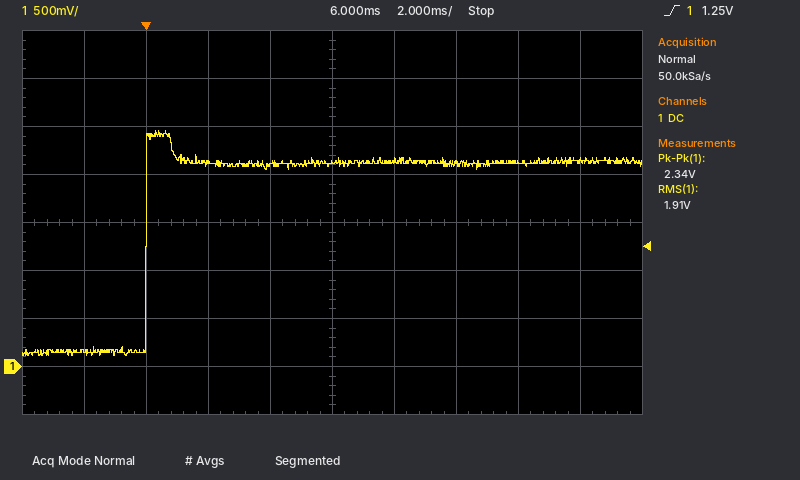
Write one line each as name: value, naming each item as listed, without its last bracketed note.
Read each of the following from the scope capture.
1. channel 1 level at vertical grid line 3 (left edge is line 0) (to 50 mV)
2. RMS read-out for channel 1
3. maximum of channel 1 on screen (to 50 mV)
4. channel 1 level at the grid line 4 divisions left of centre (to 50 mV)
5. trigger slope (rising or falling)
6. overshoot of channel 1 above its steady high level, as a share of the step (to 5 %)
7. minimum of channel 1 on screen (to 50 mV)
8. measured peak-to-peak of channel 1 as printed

channel 1 level at vertical grid line 3 (left edge is line 0): 2.10 V
RMS read-out for channel 1: 1.91 V
maximum of channel 1 on screen: 2.45 V
channel 1 level at the grid line 4 divisions left of centre: 150 mV
trigger slope: rising
overshoot of channel 1 above its steady high level, as a share of the step: 15 %
minimum of channel 1 on screen: 100 mV
measured peak-to-peak of channel 1 as printed: 2.34 V
